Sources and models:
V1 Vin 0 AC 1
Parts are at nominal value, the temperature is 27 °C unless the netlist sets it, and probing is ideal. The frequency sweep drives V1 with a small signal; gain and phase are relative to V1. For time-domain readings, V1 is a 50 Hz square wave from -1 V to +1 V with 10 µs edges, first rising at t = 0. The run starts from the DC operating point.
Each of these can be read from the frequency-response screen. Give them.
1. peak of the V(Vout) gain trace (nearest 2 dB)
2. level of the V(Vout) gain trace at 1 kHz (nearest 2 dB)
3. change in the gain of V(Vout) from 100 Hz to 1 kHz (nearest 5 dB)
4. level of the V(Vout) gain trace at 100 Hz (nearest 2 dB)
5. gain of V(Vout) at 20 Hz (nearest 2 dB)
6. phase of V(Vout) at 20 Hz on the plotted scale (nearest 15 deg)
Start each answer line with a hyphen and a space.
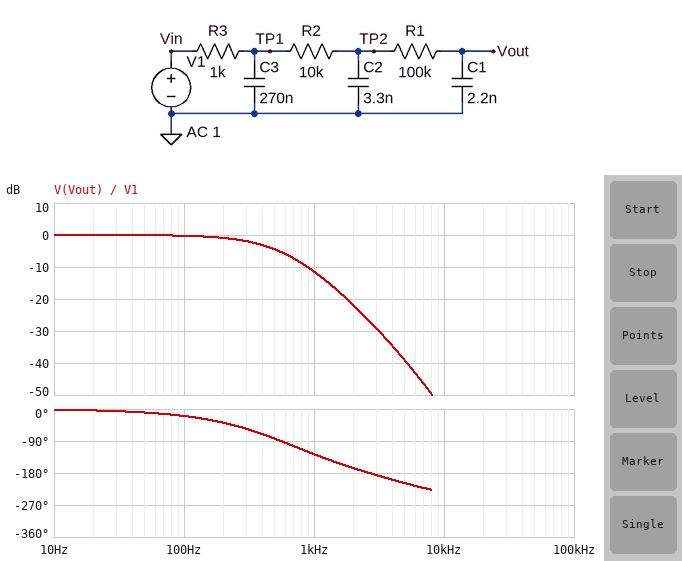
- 0 dB
- -12 dB
- -10 dB
- 0 dB
- 0 dB
- 0 deg
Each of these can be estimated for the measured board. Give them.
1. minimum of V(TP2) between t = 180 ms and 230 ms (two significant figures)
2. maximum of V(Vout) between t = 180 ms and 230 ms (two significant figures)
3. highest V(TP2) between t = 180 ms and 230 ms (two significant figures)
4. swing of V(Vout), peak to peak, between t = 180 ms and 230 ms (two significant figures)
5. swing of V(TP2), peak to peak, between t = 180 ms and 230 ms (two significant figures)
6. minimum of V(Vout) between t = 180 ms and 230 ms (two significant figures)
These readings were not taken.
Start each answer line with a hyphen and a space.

- -1.0 V
- 1.0 V
- 1.0 V
- 2.0 V
- 2.0 V
- -1.0 V
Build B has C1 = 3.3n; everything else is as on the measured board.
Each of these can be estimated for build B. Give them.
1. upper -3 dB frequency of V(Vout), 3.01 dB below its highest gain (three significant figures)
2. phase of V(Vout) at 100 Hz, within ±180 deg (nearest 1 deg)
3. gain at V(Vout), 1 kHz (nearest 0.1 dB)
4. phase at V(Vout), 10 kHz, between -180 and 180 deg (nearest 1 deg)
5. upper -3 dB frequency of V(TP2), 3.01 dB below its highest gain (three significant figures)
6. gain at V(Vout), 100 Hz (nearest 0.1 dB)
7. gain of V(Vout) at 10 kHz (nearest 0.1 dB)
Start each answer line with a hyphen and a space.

- 315 Hz
- -24 deg
- -14.1 dB
- 124 deg
- 504 Hz
- -0.4 dB
- -58.4 dB
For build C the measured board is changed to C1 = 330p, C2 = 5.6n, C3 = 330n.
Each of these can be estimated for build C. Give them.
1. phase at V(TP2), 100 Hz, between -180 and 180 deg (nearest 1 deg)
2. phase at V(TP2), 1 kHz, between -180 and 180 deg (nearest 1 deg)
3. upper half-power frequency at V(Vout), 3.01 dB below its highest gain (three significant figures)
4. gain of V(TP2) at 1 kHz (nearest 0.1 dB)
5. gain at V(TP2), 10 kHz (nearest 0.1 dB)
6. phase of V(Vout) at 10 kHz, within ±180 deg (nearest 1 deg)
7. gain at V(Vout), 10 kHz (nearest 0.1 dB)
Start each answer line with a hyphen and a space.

- -14 deg
- -85 deg
- 454 Hz
- -8.0 dB
- -37.8 dB
- 136 deg
- -45.0 dB
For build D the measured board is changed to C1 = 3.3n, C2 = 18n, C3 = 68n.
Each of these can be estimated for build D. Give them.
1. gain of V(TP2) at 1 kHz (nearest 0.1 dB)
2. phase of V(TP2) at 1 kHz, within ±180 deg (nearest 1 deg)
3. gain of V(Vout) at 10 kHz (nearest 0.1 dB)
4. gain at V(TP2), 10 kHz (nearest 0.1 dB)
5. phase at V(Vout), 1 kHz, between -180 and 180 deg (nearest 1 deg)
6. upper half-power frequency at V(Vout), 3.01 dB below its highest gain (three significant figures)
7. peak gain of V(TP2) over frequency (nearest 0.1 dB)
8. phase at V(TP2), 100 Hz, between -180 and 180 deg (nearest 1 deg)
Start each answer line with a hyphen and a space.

- -5.3 dB
- -71 deg
- -60.4 dB
- -34.0 dB
- -136 deg
- 339 Hz
- 0 dB
- -11 deg
